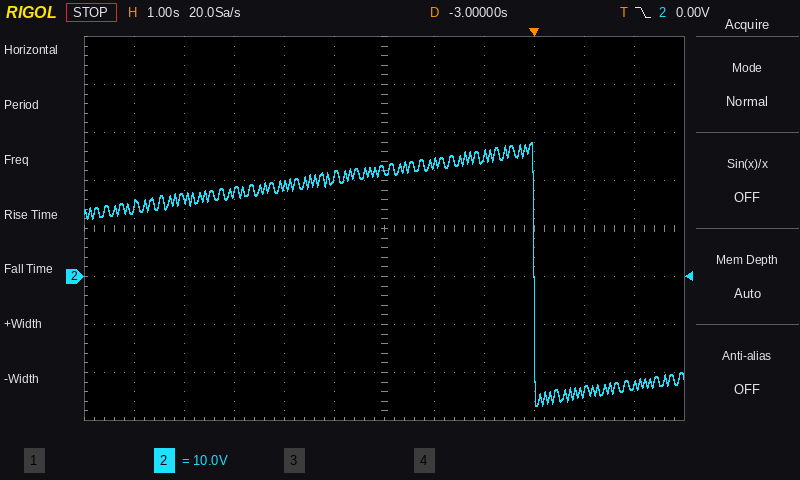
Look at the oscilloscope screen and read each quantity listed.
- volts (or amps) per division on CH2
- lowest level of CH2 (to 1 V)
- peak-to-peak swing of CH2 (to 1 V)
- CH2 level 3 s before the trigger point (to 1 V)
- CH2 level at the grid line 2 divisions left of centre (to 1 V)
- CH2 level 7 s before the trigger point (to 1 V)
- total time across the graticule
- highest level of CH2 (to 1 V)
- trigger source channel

10 V
-27 V
55 V
22 V
19 V
16 V
12 s
28 V
CH2
